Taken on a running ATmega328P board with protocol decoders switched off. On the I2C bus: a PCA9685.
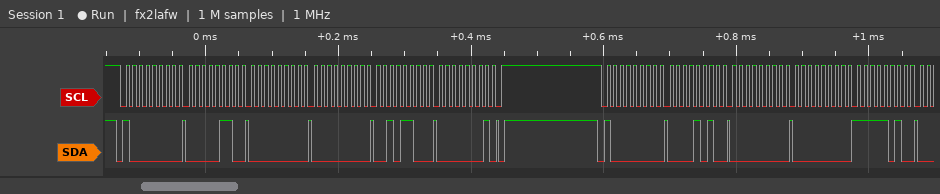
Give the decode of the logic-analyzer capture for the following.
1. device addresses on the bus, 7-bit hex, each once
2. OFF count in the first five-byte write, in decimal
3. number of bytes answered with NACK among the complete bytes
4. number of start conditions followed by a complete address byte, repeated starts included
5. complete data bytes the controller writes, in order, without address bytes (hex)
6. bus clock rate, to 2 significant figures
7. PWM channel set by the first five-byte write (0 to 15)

0x40
300
0
2
06 00 00 2C 01 0A 00 00 FA
100 kHz
0
